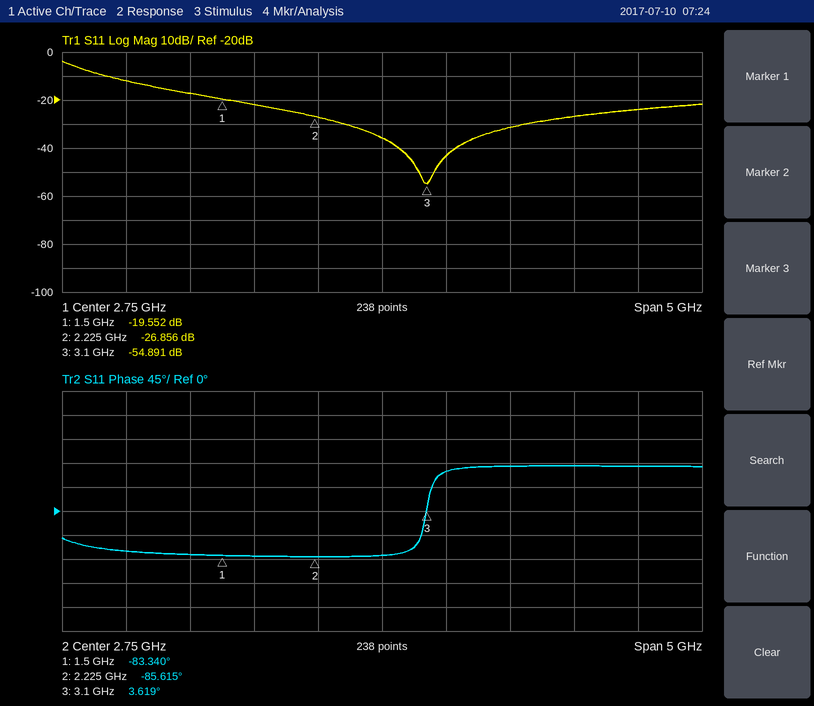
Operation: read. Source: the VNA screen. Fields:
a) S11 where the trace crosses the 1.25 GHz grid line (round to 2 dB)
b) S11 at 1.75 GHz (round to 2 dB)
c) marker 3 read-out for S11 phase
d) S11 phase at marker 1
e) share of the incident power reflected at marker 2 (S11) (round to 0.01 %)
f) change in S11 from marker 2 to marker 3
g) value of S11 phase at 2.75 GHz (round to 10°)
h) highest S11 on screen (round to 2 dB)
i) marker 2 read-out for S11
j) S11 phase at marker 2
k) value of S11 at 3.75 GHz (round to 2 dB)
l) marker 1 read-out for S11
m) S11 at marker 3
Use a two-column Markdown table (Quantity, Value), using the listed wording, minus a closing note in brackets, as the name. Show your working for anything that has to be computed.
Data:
| Quantity | Value |
|---|---|
| S11 where the trace crosses the 1.25 GHz grid line | -18 dB |
| S11 at 1.75 GHz | -22 dB |
| marker 3 read-out for S11 phase | 3.619° |
| S11 phase at marker 1 | -83.340° |
| share of the incident power reflected at marker 2 (S11) | 10^(-26.856/10) ≈ 0.21 % |
| change in S11 from marker 2 to marker 3 | -54.891 − (-26.856) = -28.035 dB |
| value of S11 phase at 2.75 GHz | -80° |
| highest S11 on screen | -4 dB |
| marker 2 read-out for S11 | -26.856 dB |
| S11 phase at marker 2 | -85.615° |
| value of S11 at 3.75 GHz | -32 dB |
| marker 1 read-out for S11 | -19.552 dB |
| S11 at marker 3 | -54.891 dB |
